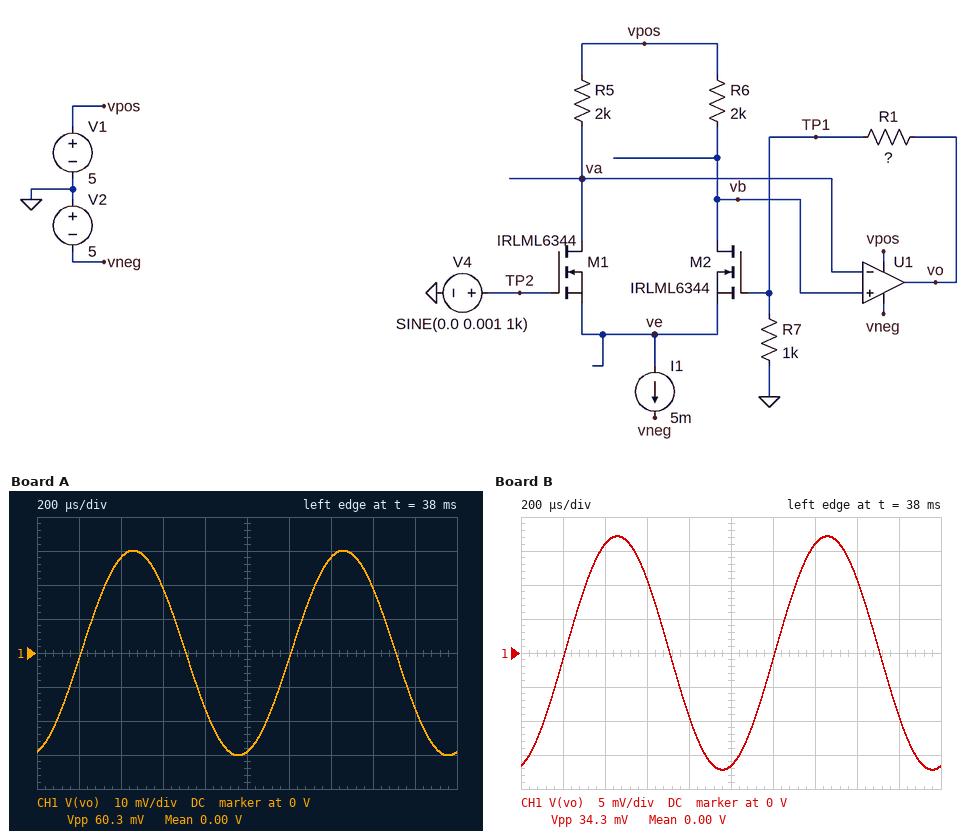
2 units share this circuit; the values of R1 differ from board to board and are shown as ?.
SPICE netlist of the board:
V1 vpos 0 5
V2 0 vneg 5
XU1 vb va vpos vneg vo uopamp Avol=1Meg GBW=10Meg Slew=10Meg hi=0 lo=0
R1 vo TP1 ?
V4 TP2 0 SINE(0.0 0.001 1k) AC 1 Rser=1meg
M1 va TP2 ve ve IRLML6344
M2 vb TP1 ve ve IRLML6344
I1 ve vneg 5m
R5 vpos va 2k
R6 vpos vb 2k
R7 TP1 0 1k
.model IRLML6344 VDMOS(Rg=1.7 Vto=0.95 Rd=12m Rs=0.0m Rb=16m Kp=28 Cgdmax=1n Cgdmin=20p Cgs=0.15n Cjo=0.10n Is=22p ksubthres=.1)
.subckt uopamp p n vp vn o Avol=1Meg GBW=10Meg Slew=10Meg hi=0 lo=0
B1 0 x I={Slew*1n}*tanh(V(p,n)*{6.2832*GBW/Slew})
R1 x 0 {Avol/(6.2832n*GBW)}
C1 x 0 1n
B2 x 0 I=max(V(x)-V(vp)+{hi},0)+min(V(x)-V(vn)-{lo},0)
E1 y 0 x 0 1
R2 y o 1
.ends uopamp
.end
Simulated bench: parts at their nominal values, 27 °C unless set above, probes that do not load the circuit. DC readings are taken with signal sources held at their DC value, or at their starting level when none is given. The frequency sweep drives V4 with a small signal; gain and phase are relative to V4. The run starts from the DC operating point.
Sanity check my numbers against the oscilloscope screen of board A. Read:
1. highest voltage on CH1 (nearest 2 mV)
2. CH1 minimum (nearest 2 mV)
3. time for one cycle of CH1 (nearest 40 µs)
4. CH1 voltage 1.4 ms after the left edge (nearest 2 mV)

30 mV
-30 mV
1.00 ms
28 mV
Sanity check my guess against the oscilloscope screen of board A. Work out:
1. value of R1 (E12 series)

120 kΩ
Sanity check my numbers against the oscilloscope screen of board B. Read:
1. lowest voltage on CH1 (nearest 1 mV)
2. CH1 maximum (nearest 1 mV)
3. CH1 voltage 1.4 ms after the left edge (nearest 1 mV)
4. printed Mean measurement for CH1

-17 mV
17 mV
16 mV
0.00 V
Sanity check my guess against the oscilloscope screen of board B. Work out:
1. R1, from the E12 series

68 kΩ
